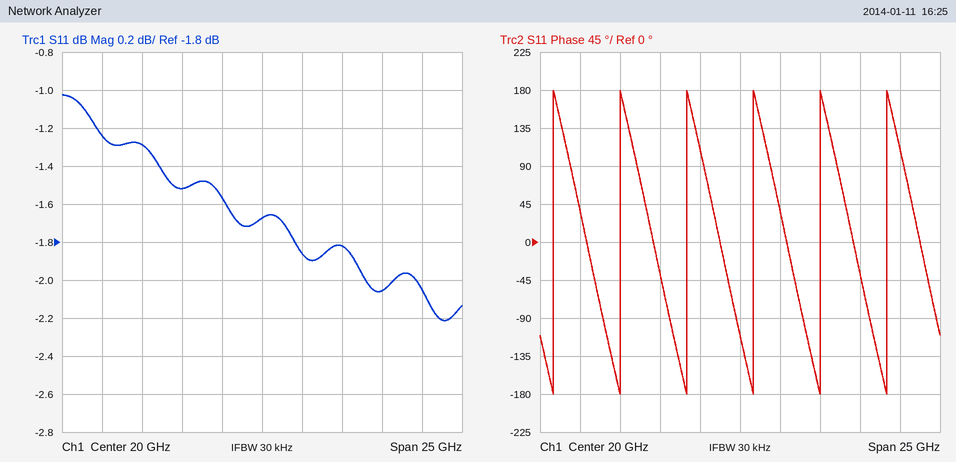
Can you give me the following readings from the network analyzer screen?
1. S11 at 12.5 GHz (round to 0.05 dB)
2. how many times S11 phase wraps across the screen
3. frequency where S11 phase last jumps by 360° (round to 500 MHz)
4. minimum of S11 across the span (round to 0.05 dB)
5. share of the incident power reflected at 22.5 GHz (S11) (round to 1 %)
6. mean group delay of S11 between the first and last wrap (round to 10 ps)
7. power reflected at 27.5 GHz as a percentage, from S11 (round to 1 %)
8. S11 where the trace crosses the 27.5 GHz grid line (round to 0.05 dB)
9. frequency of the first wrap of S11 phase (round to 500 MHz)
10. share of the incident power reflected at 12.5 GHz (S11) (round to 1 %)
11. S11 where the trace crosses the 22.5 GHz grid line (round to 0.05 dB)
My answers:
-1.30 dB
6
29.0 GHz
-2.20 dB
65 %
240 ps
62 %
-2.05 dB
8.5 GHz
74 %
-1.85 dB
